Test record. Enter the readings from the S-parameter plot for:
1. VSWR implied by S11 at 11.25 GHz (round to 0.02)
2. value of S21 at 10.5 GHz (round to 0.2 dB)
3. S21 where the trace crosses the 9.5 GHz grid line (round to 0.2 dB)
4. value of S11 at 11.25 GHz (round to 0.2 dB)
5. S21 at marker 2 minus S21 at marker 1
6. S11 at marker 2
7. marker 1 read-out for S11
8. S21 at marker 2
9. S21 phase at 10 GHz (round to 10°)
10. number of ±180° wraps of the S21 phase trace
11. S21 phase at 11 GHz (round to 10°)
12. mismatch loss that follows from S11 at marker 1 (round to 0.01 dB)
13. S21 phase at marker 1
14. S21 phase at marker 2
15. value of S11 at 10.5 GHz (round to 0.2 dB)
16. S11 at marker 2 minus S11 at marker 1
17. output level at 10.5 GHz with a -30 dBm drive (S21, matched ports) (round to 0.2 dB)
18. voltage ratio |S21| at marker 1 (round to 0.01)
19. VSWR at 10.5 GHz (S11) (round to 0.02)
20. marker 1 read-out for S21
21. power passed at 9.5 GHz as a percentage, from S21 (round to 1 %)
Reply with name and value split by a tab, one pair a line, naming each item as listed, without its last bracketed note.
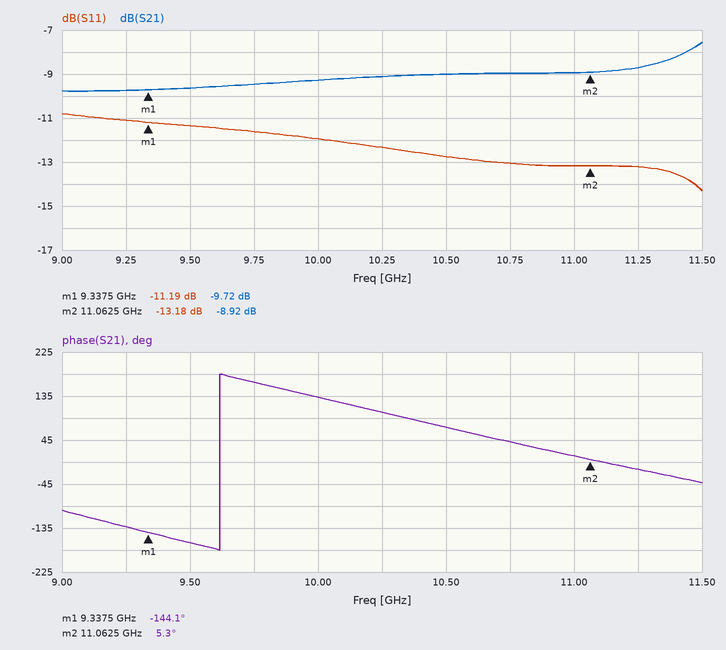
VSWR implied by S11 at 11.25 GHz	1.56
value of S21 at 10.5 GHz	-9.0 dB
S21 where the trace crosses the 9.5 GHz grid line	-9.6 dB
value of S11 at 11.25 GHz	-13.2 dB
S21 at marker 2 minus S21 at marker 1	0.80 dB
S11 at marker 2	-13.18 dB
marker 1 read-out for S11	-11.19 dB
S21 at marker 2	-8.92 dB
S21 phase at 10 GHz	130°
number of ±180° wraps of the S21 phase trace	1
S21 phase at 11 GHz	10°
mismatch loss that follows from S11 at marker 1	0.34 dB
S21 phase at marker 1	-144.1°
S21 phase at marker 2	5.3°
value of S11 at 10.5 GHz	-12.8 dB
S11 at marker 2 minus S11 at marker 1	-1.99 dB
output level at 10.5 GHz with a -30 dBm drive (S21, matched ports)	-39.0 dBm
voltage ratio |S21| at marker 1	0.33
VSWR at 10.5 GHz (S11)	1.60
marker 1 read-out for S21	-9.72 dB
power passed at 9.5 GHz as a percentage, from S21	11 %
